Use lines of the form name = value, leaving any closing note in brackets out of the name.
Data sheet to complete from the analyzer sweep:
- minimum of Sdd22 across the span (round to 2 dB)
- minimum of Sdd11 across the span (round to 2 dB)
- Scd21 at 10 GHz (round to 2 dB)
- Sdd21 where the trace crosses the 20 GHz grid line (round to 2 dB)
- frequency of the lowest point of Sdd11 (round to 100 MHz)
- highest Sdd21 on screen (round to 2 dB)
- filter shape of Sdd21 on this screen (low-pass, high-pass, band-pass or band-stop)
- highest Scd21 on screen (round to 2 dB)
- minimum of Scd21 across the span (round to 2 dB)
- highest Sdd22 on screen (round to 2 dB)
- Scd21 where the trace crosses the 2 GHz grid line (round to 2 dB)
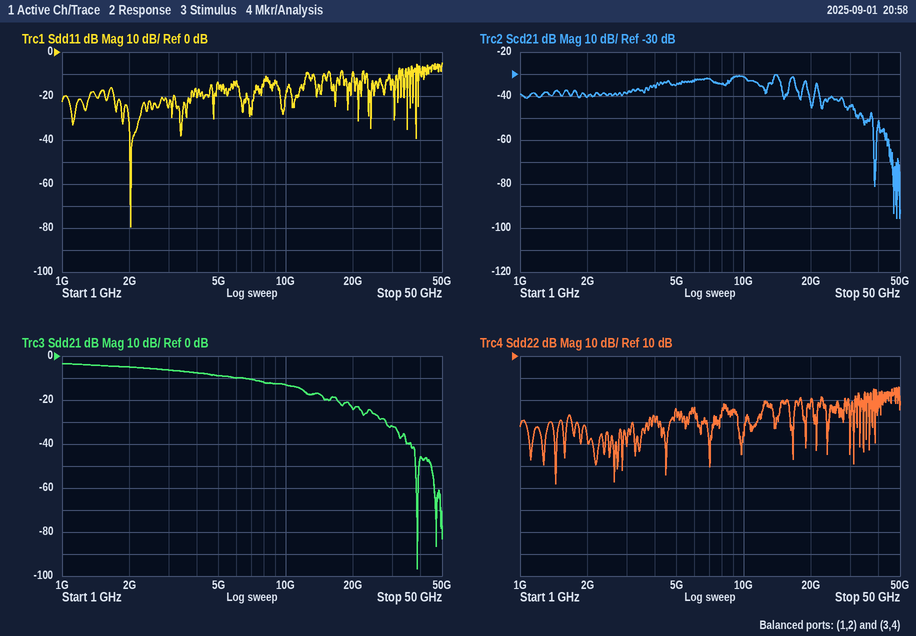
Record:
minimum of Sdd22 across the span = -48 dB
minimum of Sdd11 across the span = -80 dB
Scd21 at 10 GHz = -32 dB
Sdd21 where the trace crosses the 20 GHz grid line = -24 dB
frequency of the lowest point of Sdd11 = 2.0 GHz
highest Sdd21 on screen = -4 dB
filter shape of Sdd21 on this screen = low-pass
highest Scd21 on screen = -30 dB
minimum of Scd21 across the span = -96 dB
highest Sdd22 on screen = -4 dB
Scd21 where the trace crosses the 2 GHz grid line = -40 dB
